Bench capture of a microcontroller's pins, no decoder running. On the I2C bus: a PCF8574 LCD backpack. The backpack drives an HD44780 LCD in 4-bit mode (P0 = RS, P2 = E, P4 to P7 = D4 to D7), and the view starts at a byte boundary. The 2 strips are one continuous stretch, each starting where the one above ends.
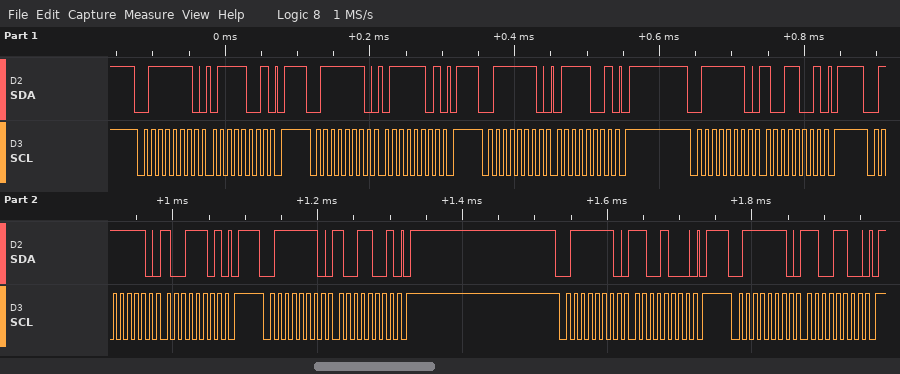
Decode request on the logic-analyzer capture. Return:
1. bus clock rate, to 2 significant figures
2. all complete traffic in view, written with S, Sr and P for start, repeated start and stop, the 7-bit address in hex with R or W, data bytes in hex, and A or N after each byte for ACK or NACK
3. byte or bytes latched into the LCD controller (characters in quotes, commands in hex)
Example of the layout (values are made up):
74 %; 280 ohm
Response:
100 kHz; S 3FW A 79 A P S 3FW A 7D A P S 3FW A 79 A P S 3FW A 99 A P S 3FW A 9D A P S 3FW A 99 A P S 3FW A C8 A P S 3FW A CC A P; 'y'
